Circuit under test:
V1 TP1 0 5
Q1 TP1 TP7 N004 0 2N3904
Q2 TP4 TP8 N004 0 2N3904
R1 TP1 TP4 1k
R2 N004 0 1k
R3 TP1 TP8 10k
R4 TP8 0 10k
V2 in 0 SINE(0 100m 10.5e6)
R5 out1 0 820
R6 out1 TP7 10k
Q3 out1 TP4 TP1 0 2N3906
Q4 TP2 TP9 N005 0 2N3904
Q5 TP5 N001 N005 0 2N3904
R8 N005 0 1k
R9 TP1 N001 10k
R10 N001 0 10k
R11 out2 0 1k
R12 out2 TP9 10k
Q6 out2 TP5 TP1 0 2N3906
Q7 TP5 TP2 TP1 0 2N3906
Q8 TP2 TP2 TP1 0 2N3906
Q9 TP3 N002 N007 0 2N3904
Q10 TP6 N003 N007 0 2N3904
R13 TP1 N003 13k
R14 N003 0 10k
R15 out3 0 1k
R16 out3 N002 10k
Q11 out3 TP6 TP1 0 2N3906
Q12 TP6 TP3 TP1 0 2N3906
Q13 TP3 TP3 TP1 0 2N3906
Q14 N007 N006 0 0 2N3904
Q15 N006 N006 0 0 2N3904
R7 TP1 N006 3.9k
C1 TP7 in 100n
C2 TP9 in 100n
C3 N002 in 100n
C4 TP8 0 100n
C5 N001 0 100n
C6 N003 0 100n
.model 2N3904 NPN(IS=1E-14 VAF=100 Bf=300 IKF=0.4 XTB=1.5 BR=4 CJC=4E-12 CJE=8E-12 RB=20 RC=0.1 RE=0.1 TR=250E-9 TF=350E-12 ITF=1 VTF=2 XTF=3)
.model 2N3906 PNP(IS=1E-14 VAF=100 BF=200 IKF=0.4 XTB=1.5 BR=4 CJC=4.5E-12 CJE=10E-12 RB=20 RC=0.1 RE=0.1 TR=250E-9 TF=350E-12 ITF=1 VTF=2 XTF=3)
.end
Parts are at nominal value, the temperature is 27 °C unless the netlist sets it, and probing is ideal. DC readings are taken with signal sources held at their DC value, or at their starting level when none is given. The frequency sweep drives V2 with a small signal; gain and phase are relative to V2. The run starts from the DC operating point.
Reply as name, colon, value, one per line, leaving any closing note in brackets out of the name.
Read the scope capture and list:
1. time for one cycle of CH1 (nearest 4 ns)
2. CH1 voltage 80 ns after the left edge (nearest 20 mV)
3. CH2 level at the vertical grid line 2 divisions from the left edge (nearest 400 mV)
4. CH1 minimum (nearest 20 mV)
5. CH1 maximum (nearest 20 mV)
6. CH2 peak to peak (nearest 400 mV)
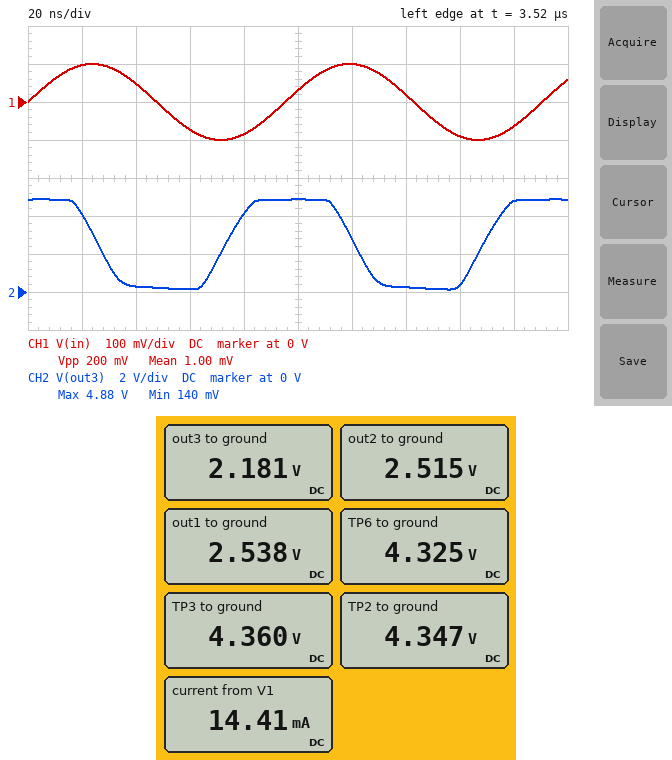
time for one cycle of CH1: 96 ns
CH1 voltage 80 ns after the left edge: -80 mV
CH2 level at the vertical grid line 2 divisions from the left edge: 400 mV
CH1 minimum: -100 mV
CH1 maximum: 100 mV
CH2 peak to peak: 4.8 V
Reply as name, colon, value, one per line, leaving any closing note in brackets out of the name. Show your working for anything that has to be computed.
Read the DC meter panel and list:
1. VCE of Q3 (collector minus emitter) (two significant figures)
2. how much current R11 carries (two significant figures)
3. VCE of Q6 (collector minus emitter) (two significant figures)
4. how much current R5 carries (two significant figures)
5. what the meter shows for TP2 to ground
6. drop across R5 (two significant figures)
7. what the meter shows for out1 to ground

VCE of Q3 (collector minus emitter): 2.538 V - 5 V = -2.5 V
how much current R11 carries: (2.515 V) / 1 kΩ = 2.5 mA
VCE of Q6 (collector minus emitter): 2.515 V - 5 V = -2.5 V
how much current R5 carries: (2.538 V) / 820 Ω = 3.1 mA
what the meter shows for TP2 to ground: 4.347 V
drop across R5: 2.538 V = 2.5 V
what the meter shows for out1 to ground: 2.538 V
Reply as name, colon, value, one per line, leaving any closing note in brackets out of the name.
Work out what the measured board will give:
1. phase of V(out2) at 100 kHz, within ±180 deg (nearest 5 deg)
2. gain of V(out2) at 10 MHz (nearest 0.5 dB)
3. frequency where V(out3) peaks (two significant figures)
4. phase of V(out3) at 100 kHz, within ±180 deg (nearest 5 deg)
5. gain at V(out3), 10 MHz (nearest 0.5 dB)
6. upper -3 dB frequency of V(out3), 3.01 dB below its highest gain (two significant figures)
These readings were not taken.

phase of V(out2) at 100 kHz, within ±180 deg: -95 deg
gain of V(out2) at 10 MHz: 43.0 dB
frequency where V(out3) peaks: 380 kHz
phase of V(out3) at 100 kHz, within ±180 deg: -100 deg
gain at V(out3), 10 MHz: 39.0 dB
upper -3 dB frequency of V(out3), 3.01 dB below its highest gain: 520 kHz
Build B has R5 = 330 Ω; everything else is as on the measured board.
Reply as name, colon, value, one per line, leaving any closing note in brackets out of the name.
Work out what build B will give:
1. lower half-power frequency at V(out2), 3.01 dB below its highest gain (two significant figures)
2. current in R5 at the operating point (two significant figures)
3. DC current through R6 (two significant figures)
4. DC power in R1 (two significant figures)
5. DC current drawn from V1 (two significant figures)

lower half-power frequency at V(out2), 3.01 dB below its highest gain: 380 kHz
current in R5 at the operating point: 7.7 mA
DC current through R6: 3.5 µA
DC power in R1: 500 µW
DC current drawn from V1: 19 mA
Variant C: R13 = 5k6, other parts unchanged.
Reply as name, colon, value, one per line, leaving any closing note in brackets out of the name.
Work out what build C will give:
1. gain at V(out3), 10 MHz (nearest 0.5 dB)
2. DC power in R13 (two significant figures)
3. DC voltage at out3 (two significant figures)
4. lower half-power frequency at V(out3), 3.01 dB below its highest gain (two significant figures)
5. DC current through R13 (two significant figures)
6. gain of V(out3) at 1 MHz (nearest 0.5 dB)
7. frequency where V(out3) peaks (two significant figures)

gain at V(out3), 10 MHz: 38.5 dB
DC power in R13: 580 µW
DC voltage at out3: 3.2 V
lower half-power frequency at V(out3), 3.01 dB below its highest gain: 270 kHz
DC current through R13: 320 µA
gain of V(out3) at 1 MHz: 59.5 dB
frequency where V(out3) peaks: 370 kHz
